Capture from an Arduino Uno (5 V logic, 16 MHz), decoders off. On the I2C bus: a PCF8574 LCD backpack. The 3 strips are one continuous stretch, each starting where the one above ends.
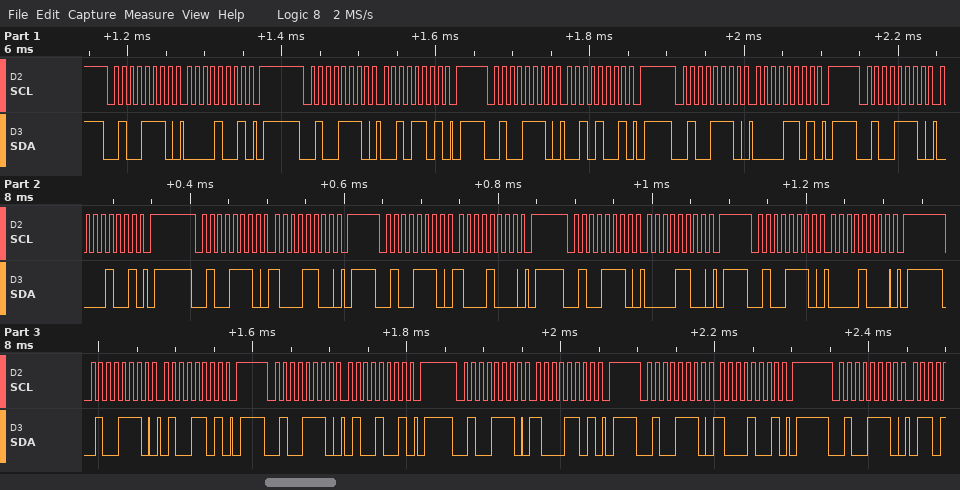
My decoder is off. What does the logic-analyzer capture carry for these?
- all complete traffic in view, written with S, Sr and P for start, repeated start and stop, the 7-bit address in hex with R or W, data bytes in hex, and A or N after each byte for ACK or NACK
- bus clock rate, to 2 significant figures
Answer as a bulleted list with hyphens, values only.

- S 27W A 09 A P S 27W A 2D A P S 27W A 29 A P S 27W A 0D A P S 27W A 09 A P S 27W A 8C A P S 27W A 88 A P S 27W A 0C A P S 27W A 08 A P S 27W A 4D A P S 27W A 49 A P S 27W A 8D A P S 27W A 89 A P S 27W A
- 100 kHz
